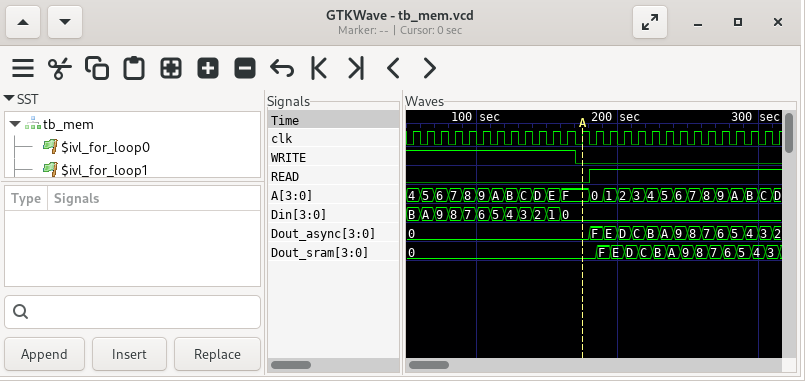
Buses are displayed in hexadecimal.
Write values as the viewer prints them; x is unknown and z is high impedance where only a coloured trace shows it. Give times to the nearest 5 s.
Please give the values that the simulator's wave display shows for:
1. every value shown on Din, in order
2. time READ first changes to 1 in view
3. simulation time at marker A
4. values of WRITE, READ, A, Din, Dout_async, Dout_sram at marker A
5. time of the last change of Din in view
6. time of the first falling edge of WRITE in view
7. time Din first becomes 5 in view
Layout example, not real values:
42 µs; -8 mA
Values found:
B, A, 9, 8, 7, 6, 5, 4, 3, 2, 1, 0; 180 s; 175 s; WRITE=0, READ=0, A=F, Din=0, Dout_async=0, Dout_sram=0; 160 s; 170 s; 110 s
